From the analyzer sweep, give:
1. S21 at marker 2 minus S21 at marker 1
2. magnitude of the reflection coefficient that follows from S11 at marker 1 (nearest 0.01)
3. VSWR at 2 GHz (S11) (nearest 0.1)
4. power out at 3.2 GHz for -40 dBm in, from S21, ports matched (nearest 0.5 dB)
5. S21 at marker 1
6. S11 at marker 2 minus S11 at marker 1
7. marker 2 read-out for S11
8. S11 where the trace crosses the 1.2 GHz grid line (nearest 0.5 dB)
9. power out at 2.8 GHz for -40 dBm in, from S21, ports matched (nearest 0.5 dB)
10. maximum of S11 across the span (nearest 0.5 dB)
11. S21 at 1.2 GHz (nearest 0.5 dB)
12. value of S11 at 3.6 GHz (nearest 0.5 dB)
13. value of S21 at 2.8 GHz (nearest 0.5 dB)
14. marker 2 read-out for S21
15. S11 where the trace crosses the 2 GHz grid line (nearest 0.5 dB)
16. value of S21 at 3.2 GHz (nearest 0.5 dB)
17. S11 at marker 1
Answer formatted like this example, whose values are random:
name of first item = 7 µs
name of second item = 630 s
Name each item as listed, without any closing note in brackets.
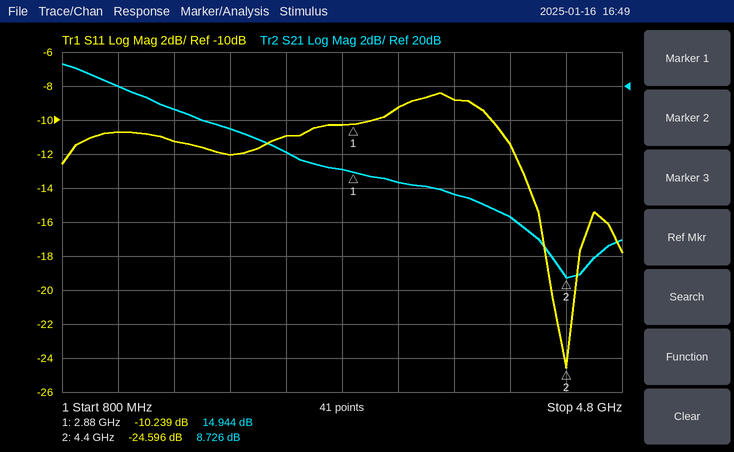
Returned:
S21 at marker 2 minus S21 at marker 1 = -6.218 dB
magnitude of the reflection coefficient that follows from S11 at marker 1 = 0.31
VSWR at 2 GHz (S11) = 1.7
power out at 3.2 GHz for -40 dBm in, from S21, ports matched = -25.5 dBm
S21 at marker 1 = 14.944 dB
S11 at marker 2 minus S11 at marker 1 = -14.357 dB
marker 2 read-out for S11 = -24.596 dB
S11 where the trace crosses the 1.2 GHz grid line = -10.5 dB
power out at 2.8 GHz for -40 dBm in, from S21, ports matched = -25.0 dBm
maximum of S11 across the span = -8.5 dB
S21 at 1.2 GHz = 20.0 dB
value of S11 at 3.6 GHz = -9.0 dB
value of S21 at 2.8 GHz = 15.0 dB
marker 2 read-out for S21 = 8.726 dB
S11 where the trace crosses the 2 GHz grid line = -12.0 dB
value of S21 at 3.2 GHz = 14.5 dB
S11 at marker 1 = -10.239 dB
